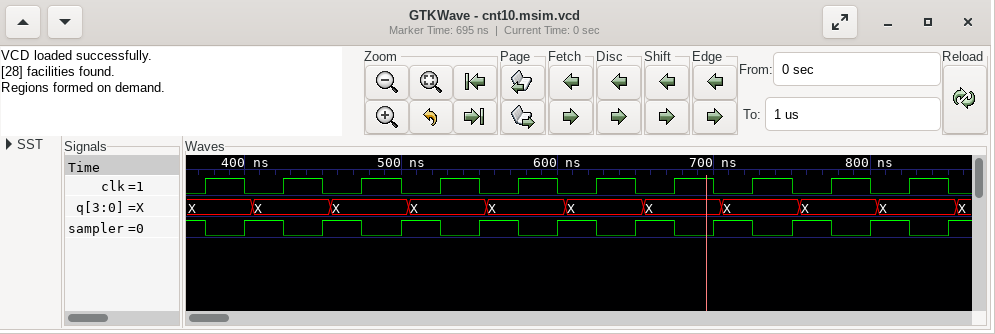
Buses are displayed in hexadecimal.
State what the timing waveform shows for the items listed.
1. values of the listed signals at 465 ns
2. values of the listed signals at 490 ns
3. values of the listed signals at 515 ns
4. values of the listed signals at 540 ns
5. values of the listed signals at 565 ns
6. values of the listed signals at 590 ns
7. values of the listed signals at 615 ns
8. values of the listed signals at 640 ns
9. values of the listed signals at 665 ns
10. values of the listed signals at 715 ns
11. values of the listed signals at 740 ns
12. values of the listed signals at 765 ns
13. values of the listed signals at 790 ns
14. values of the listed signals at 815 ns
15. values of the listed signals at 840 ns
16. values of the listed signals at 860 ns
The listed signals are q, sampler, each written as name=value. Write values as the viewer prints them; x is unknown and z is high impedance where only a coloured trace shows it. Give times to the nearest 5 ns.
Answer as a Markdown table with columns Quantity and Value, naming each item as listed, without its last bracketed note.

| Quantity | Value |
|---|---|
| values of the listed signals at 465 ns | q=X, sampler=1 |
| values of the listed signals at 490 ns | q=X, sampler=0 |
| values of the listed signals at 515 ns | q=X, sampler=1 |
| values of the listed signals at 540 ns | q=X, sampler=0 |
| values of the listed signals at 565 ns | q=X, sampler=1 |
| values of the listed signals at 590 ns | q=X, sampler=0 |
| values of the listed signals at 615 ns | q=X, sampler=1 |
| values of the listed signals at 640 ns | q=X, sampler=0 |
| values of the listed signals at 665 ns | q=X, sampler=1 |
| values of the listed signals at 715 ns | q=X, sampler=1 |
| values of the listed signals at 740 ns | q=X, sampler=0 |
| values of the listed signals at 765 ns | q=X, sampler=1 |
| values of the listed signals at 790 ns | q=X, sampler=0 |
| values of the listed signals at 815 ns | q=X, sampler=1 |
| values of the listed signals at 840 ns | q=X, sampler=0 |
| values of the listed signals at 860 ns | q=X, sampler=1 |
